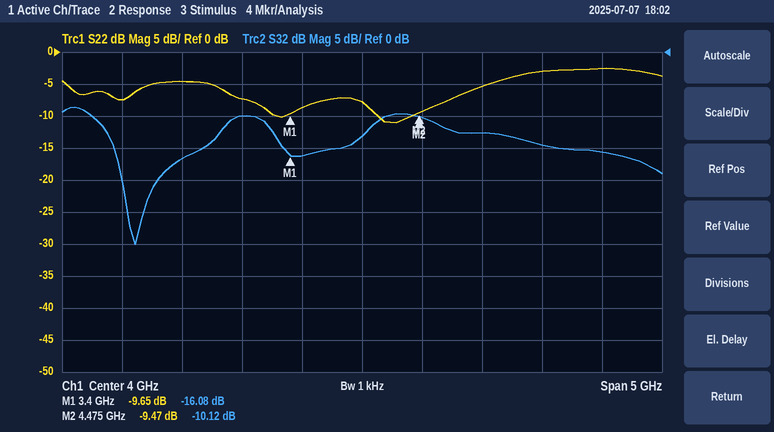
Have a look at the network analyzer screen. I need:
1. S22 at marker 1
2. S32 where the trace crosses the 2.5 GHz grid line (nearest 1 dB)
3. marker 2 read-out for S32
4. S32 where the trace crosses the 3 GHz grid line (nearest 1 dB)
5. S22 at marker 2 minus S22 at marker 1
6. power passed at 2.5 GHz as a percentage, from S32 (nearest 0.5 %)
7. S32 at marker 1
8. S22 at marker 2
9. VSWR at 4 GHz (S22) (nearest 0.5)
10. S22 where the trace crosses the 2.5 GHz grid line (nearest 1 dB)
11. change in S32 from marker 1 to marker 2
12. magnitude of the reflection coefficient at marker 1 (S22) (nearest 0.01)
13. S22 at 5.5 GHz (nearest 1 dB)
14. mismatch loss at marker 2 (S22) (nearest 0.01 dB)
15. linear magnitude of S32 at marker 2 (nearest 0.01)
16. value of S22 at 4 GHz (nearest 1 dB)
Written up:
-9.65 dB
-17 dB
-10.12 dB
-10 dB
0.18 dB
2.0 %
-16.08 dB
-9.47 dB
2.5
-5 dB
5.96 dB
0.33
-3 dB
0.52 dB
0.31
-8 dB
